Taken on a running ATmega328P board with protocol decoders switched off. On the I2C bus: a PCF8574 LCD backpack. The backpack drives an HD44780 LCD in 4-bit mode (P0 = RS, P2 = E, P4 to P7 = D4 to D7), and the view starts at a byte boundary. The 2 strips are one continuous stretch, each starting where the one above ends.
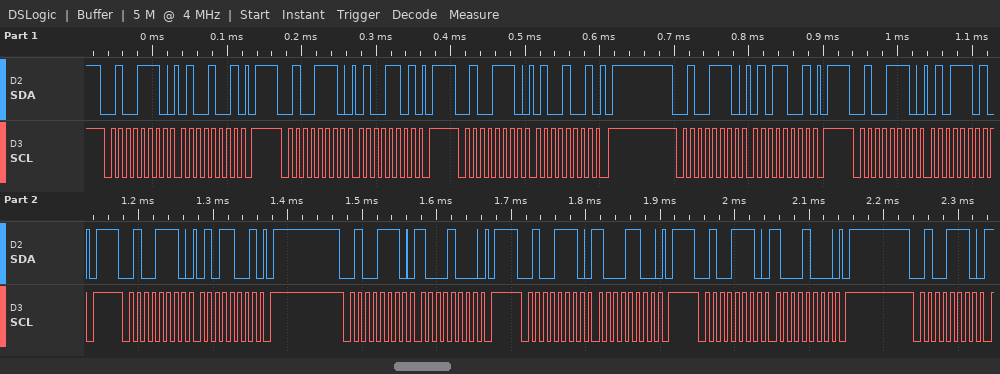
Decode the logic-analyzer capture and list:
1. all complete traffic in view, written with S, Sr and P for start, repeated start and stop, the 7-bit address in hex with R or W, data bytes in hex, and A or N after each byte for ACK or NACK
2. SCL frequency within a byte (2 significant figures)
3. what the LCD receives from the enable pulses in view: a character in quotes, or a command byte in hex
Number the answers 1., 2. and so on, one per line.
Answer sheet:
1. S 27W A 49 A P S 27W A 4D A P S 27W A 49 A P S 27W A 59 A P S 27W A 5D A P S 27W A 59 A P S 27W A 88 A P S 27W A 8C A P S 27W A 88 A P S 27W A
2. 100 kHz
3. 'E'
